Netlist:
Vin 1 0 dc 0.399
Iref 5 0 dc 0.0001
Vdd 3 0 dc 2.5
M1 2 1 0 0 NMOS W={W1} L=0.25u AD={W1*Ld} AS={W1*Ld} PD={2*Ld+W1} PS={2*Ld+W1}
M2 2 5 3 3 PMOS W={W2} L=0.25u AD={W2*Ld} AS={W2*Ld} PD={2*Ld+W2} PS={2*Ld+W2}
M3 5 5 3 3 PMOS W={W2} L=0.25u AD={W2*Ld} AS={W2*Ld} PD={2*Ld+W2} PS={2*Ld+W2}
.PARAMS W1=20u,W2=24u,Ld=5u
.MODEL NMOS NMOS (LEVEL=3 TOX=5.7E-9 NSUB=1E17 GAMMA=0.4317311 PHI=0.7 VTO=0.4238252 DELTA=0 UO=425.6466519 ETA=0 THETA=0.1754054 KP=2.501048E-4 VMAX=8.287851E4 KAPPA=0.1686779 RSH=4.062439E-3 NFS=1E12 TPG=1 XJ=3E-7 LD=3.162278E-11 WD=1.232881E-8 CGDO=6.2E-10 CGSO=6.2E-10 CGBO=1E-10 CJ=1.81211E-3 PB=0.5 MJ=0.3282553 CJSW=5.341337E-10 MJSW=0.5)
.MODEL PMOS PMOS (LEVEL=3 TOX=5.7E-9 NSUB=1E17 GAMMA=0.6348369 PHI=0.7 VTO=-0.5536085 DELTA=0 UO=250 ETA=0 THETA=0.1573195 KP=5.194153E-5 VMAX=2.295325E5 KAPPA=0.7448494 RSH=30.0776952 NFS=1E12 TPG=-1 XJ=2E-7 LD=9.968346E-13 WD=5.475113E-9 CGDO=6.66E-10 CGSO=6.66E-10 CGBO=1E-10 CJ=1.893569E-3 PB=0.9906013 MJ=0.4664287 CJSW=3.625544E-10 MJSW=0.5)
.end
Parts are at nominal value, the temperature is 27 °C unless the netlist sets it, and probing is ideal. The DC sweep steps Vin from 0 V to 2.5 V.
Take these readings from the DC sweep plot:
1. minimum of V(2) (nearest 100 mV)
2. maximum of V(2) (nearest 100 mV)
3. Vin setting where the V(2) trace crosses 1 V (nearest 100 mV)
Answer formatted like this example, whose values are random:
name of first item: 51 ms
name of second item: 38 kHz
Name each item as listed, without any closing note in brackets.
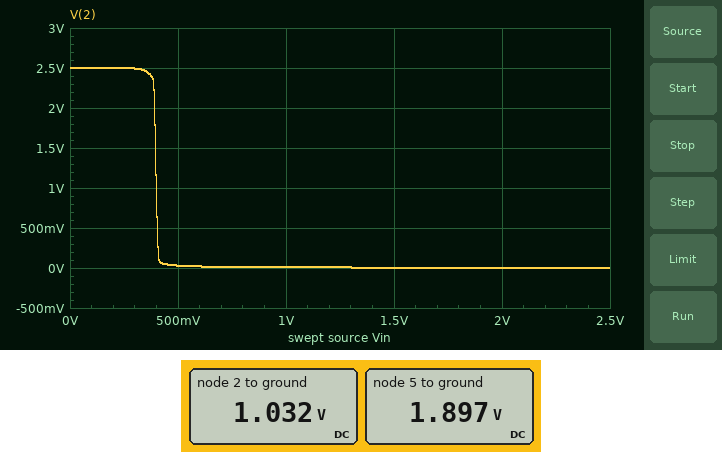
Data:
minimum of V(2): 0 V
maximum of V(2): 2.5 V
Vin setting where the V(2) trace crosses 1 V: 400 mV
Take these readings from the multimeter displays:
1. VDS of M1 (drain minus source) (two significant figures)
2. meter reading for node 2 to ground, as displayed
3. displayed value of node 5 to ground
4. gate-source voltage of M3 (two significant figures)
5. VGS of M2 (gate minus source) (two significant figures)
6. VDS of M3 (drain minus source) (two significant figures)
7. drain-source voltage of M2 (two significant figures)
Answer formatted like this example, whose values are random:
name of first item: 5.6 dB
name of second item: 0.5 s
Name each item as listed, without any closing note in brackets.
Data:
VDS of M1 (drain minus source): 1.0 V
meter reading for node 2 to ground, as displayed: 1.032 V
displayed value of node 5 to ground: 1.897 V
gate-source voltage of M3: -600 mV
VGS of M2 (gate minus source): -600 mV
VDS of M3 (drain minus source): -600 mV
drain-source voltage of M2: -1.5 V
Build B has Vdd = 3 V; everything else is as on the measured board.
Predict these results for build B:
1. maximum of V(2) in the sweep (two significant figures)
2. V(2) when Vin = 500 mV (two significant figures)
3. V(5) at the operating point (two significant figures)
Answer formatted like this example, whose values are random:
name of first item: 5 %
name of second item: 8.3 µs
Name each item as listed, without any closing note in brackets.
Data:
maximum of V(2) in the sweep: 3.0 V
V(2) when Vin = 500 mV: 31 mV
V(5) at the operating point: 2.4 V
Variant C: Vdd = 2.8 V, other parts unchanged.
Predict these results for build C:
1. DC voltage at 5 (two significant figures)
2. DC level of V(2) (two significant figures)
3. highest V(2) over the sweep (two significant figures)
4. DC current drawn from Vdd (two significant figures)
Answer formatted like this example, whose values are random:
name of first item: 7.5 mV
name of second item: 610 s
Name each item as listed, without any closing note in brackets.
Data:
DC voltage at 5: 2.2 V
DC level of V(2): 1.1 V
highest V(2) over the sweep: 2.8 V
DC current drawn from Vdd: 200 µA
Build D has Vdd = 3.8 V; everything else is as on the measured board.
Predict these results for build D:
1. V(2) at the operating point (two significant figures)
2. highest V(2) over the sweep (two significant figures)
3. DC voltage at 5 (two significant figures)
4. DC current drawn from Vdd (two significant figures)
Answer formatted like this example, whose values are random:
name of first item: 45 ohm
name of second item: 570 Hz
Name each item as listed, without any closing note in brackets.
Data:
V(2) at the operating point: 1.3 V
highest V(2) over the sweep: 3.8 V
DC voltage at 5: 3.2 V
DC current drawn from Vdd: 210 µA
